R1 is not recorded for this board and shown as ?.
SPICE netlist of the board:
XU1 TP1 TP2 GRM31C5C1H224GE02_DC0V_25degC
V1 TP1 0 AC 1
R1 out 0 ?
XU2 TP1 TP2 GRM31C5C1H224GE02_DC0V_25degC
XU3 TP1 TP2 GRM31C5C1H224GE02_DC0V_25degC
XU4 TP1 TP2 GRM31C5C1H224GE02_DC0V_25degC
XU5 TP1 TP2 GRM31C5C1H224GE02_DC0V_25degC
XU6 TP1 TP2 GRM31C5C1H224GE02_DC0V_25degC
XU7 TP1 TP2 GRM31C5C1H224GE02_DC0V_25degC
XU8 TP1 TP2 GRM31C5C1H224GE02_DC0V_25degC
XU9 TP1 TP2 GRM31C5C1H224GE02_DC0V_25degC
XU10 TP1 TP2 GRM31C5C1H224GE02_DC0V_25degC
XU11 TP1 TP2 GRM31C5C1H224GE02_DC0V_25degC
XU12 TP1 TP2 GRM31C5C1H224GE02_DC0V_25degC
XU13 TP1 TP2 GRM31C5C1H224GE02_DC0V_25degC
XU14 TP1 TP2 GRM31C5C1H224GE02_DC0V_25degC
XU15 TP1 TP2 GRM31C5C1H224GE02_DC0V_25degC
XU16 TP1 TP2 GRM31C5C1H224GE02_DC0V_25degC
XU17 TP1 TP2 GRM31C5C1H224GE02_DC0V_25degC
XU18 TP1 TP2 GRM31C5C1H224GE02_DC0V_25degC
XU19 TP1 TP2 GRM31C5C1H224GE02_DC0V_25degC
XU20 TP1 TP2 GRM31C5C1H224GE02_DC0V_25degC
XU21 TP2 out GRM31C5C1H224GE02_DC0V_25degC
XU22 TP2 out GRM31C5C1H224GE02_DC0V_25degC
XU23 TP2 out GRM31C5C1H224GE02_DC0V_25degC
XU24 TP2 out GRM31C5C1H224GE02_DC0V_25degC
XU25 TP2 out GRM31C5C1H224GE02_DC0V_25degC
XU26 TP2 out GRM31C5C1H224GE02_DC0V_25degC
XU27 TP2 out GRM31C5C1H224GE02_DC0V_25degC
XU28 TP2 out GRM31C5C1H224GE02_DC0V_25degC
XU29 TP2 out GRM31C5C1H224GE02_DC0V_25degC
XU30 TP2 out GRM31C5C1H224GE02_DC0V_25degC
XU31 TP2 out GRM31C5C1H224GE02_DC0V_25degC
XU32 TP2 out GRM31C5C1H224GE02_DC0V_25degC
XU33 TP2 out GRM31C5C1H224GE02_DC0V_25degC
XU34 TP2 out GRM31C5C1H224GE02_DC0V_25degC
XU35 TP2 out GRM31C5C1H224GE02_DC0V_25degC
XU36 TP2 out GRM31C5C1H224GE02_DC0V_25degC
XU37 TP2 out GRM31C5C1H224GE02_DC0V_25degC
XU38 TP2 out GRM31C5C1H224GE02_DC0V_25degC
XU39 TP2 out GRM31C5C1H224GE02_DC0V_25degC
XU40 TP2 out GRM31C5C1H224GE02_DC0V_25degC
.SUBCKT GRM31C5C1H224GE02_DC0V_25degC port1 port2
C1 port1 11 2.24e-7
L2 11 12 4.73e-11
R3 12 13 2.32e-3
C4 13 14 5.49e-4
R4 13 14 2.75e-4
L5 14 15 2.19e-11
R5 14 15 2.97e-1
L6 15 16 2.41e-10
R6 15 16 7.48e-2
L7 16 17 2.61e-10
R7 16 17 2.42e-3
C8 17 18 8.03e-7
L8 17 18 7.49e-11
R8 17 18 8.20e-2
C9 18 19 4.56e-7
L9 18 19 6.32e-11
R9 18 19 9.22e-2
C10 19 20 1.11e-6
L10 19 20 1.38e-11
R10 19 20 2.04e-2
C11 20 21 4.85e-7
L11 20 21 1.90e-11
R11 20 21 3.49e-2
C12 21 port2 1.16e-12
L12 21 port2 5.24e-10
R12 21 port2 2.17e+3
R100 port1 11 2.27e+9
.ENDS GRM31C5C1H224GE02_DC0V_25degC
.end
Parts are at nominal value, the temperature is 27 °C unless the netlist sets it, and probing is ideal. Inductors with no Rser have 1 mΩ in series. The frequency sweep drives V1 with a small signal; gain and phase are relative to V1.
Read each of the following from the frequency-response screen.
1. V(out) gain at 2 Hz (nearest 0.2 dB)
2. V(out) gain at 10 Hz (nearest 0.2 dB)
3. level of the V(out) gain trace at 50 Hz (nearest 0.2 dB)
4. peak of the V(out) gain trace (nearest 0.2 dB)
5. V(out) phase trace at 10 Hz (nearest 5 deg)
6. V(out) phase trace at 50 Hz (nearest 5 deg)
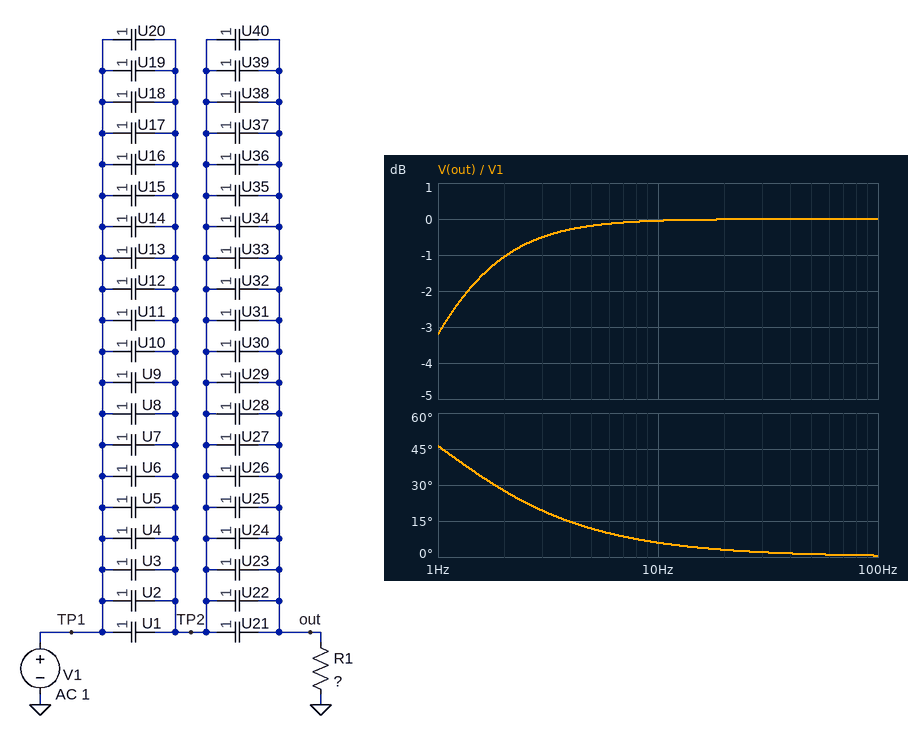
-1.0 dB
0 dB
0 dB
0 dB
5 deg
0 deg
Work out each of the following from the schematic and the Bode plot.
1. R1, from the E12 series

68 kΩ
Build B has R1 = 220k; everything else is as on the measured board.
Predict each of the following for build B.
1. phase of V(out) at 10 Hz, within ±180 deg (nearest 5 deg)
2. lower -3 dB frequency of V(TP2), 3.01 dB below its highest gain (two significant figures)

0 deg
230 mHz
